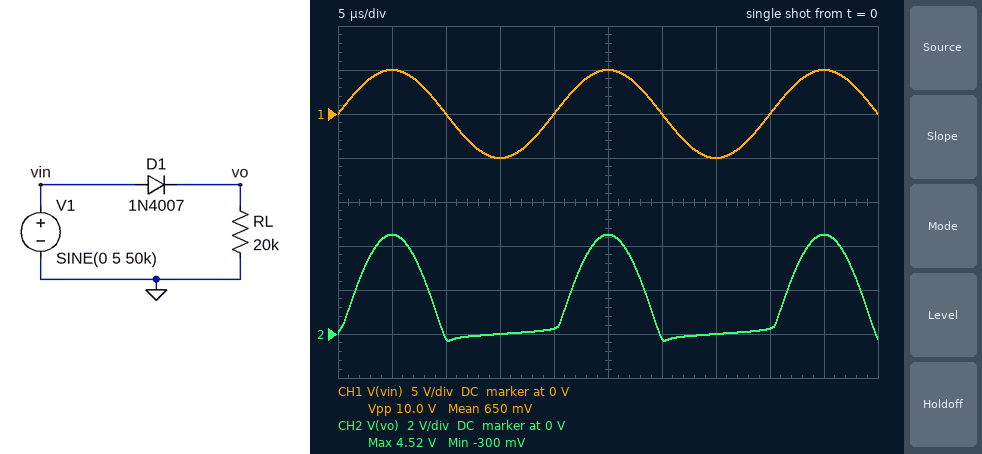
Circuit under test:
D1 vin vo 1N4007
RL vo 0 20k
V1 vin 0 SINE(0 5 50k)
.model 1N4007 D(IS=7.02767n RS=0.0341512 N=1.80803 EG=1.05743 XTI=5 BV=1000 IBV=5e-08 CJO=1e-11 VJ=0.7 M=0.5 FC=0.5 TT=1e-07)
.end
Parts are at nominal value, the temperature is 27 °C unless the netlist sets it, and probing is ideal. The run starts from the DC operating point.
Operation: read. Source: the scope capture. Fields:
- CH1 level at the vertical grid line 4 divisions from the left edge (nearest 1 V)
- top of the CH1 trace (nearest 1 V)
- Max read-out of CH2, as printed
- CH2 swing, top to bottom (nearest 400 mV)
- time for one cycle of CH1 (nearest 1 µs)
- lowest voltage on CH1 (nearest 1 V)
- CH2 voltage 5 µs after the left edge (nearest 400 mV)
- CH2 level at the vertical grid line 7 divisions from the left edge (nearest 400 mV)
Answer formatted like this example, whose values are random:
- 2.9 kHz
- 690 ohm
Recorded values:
- 0 V
- 5 V
- 4.52 V
- 4.8 V
- 20 µs
- -5 V
- 4.4 V
- 0 V
